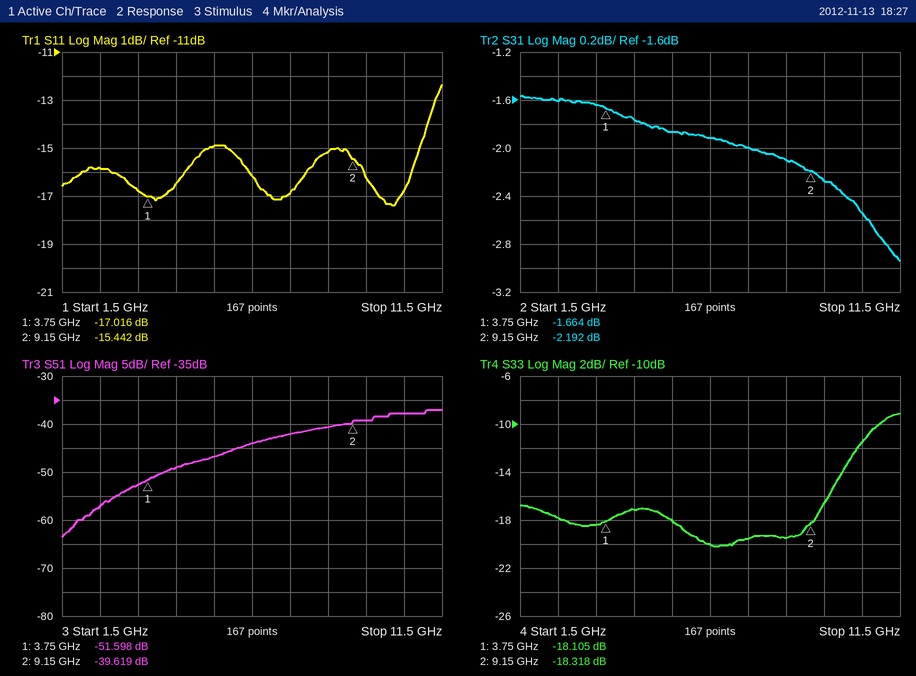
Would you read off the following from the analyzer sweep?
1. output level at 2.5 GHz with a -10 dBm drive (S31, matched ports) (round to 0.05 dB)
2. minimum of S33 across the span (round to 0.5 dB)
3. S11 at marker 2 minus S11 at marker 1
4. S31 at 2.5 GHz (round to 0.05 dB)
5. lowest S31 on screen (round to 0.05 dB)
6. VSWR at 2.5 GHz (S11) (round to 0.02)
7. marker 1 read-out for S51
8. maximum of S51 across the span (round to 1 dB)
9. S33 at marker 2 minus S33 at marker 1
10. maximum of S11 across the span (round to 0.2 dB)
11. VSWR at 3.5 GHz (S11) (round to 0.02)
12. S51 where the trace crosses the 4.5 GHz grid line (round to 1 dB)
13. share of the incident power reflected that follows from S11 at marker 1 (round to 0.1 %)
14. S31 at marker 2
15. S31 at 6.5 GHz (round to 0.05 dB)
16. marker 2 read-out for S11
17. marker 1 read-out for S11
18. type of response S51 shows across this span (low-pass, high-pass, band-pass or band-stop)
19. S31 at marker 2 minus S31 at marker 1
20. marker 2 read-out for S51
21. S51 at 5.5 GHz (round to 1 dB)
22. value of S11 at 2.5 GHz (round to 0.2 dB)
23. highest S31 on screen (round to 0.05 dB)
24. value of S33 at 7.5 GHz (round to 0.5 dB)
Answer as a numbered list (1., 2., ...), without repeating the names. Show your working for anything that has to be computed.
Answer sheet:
1. -10 dBm + (-1.60 dB) = -11.60 dBm
2. -20.0 dB
3. -15.442 − (-17.016) = 1.574 dB
4. -1.60 dB
5. -2.95 dB
6. |Γ| = 10^(-15.8/20) = 0.1622; VSWR = (1 + 0.1622)/(1 − 0.1622) ≈ 1.39, so 1.38 to the nearest 0.02
7. -51.598 dB
8. -37 dB
9. -18.318 − (-18.105) = -0.213 dB
10. -12.4 dB
11. |Γ| = 10^(-16.8/20) = 0.1445; VSWR = (1 + 0.1445)/(1 − 0.1445) ≈ 1.34
12. -49 dB
13. 10^(-17.016/10) ≈ 2.0 %
14. -2.192 dB
15. -1.90 dB
16. -15.442 dB
17. -17.016 dB
18. high-pass
19. -2.192 − (-1.664) = -0.528 dB
20. -39.619 dB
21. -47 dB
22. -15.8 dB
23. -1.55 dB
24. -19.5 dB
